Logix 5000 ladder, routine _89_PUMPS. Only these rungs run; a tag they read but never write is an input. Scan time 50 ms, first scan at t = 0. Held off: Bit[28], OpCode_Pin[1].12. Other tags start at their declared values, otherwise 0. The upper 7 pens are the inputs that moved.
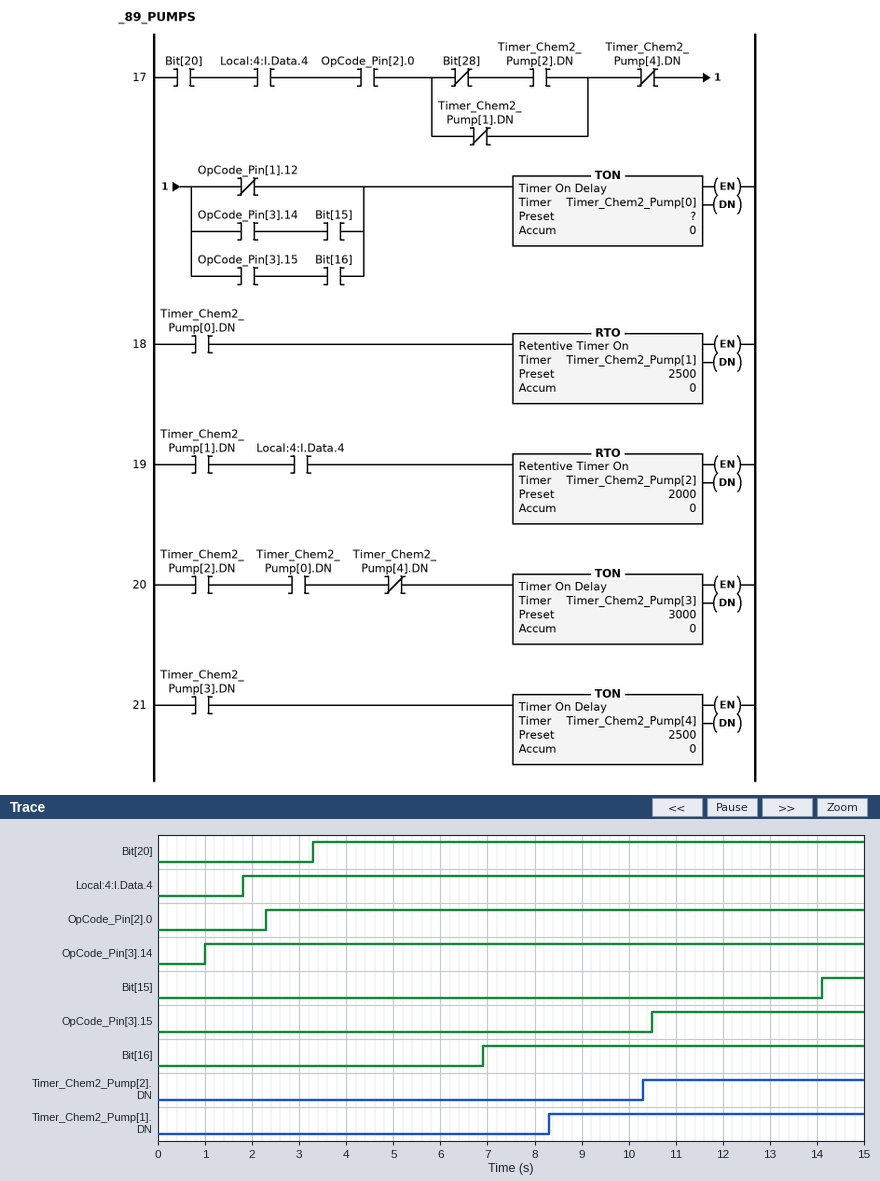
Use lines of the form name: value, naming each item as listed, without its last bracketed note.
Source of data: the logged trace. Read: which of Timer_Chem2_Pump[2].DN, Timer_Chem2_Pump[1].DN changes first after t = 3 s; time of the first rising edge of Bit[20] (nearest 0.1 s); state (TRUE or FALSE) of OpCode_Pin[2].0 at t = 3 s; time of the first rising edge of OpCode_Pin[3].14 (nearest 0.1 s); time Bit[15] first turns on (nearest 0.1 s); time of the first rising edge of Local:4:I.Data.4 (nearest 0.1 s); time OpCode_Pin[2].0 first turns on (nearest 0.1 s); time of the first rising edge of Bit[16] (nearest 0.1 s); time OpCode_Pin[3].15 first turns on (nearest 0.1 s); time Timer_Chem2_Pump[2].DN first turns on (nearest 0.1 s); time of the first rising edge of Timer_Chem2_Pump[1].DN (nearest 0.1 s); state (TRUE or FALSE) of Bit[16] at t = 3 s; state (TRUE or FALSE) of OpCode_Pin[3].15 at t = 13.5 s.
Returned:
which of Timer_Chem2_Pump[2].DN, Timer_Chem2_Pump[1].DN changes first after t = 3 s: Timer_Chem2_Pump[1].DN
time of the first rising edge of Bit[20]: 3.3 s
state (TRUE or FALSE) of OpCode_Pin[2].0 at t = 3 s: TRUE
time of the first rising edge of OpCode_Pin[3].14: 1.0 s
time Bit[15] first turns on: 14.1 s
time of the first rising edge of Local:4:I.Data.4: 1.8 s
time OpCode_Pin[2].0 first turns on: 2.3 s
time of the first rising edge of Bit[16]: 6.9 s
time OpCode_Pin[3].15 first turns on: 10.5 s
time Timer_Chem2_Pump[2].DN first turns on: 10.3 s
time of the first rising edge of Timer_Chem2_Pump[1].DN: 8.3 s
state (TRUE or FALSE) of Bit[16] at t = 3 s: FALSE
state (TRUE or FALSE) of OpCode_Pin[3].15 at t = 13.5 s: TRUE
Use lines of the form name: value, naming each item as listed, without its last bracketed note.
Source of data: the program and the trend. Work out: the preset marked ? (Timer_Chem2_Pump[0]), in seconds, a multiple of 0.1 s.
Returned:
the preset marked ? (Timer_Chem2_Pump[0]), in seconds, a multiple of 0.1 s: 2.5 s
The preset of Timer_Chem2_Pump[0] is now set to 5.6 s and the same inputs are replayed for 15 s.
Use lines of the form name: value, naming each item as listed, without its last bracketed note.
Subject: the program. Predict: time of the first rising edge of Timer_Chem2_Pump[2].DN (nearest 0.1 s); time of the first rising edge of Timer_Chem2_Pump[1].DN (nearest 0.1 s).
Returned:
time of the first rising edge of Timer_Chem2_Pump[2].DN: 13.4 s
time of the first rising edge of Timer_Chem2_Pump[1].DN: 11.4 s
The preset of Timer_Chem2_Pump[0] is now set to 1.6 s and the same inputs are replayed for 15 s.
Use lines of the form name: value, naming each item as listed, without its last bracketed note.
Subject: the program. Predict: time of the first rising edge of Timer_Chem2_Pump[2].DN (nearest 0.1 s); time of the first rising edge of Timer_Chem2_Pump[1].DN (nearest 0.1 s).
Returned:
time of the first rising edge of Timer_Chem2_Pump[2].DN: 9.4 s
time of the first rising edge of Timer_Chem2_Pump[1].DN: 7.4 s
